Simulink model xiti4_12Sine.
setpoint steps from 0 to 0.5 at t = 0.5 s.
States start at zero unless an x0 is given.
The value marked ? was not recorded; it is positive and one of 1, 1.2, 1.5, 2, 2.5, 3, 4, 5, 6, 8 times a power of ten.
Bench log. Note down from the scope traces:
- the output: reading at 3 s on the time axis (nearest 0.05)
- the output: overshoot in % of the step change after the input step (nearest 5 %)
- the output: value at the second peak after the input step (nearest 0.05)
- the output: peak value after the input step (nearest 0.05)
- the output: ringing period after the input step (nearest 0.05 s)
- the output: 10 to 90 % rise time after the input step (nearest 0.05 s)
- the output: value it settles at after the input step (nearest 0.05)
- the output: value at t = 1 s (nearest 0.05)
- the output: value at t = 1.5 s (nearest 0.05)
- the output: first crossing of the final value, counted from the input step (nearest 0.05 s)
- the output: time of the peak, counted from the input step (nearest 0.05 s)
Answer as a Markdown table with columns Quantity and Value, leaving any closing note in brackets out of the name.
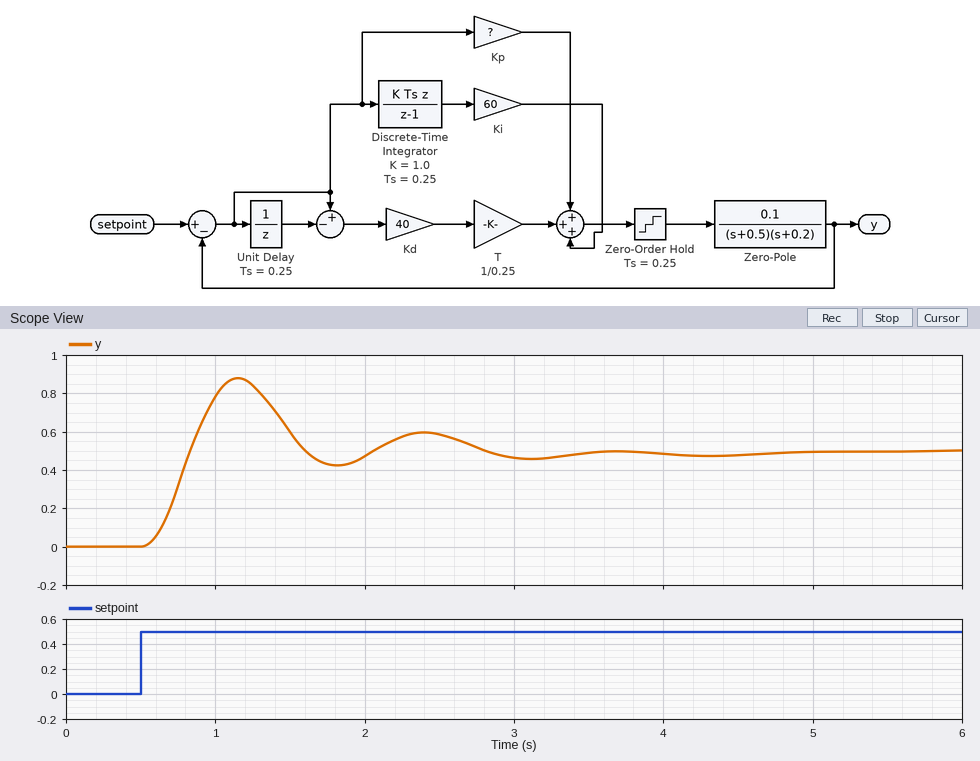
| Quantity | Value |
|---|---|
| the output: reading at 3 s on the time axis | 0.45 |
| the output: overshoot in % of the step change after the input step | 75 % |
| the output: value at the second peak after the input step | 0.60 |
| the output: peak value after the input step | 0.90 |
| the output: ringing period after the input step | 1.25 s |
| the output: 10 to 90 % rise time after the input step | 0.20 s |
| the output: value it settles at after the input step | 0.50 |
| the output: value at t = 1 s | 0.80 |
| the output: value at t = 1.5 s | 0.60 |
| the output: first crossing of the final value, counted from the input step | 0.35 s |
| the output: time of the peak, counted from the input step | 0.65 s |
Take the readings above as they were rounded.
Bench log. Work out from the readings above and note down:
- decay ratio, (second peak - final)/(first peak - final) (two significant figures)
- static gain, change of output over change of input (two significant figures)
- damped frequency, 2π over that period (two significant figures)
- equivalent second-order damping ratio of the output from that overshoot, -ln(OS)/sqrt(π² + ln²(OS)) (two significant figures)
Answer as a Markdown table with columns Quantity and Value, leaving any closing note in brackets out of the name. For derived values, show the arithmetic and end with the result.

| Quantity | Value |
|---|---|
| decay ratio, (second peak - final)/(first peak - final) | (0.6 - 0.5) / (0.9 - 0.5) = 0.25 |
| static gain, change of output over change of input | (0.5 - 0) / (0.5 - 0) = 1.0 |
| damped frequency, 2π over that period | 2π / 1.25 = 5.0 rad/s |
| equivalent second-order damping ratio of the output from that overshoot, -ln(OS)/sqrt(π² + ln²(OS)) | ln(0.75) = -0.288; 0.288 / sqrt(9.870 + 0.083) = 0.091 |
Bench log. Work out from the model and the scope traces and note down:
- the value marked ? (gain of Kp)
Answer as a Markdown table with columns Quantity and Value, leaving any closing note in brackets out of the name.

| Quantity | Value |
|---|---|
| the value marked ? | 40 |
